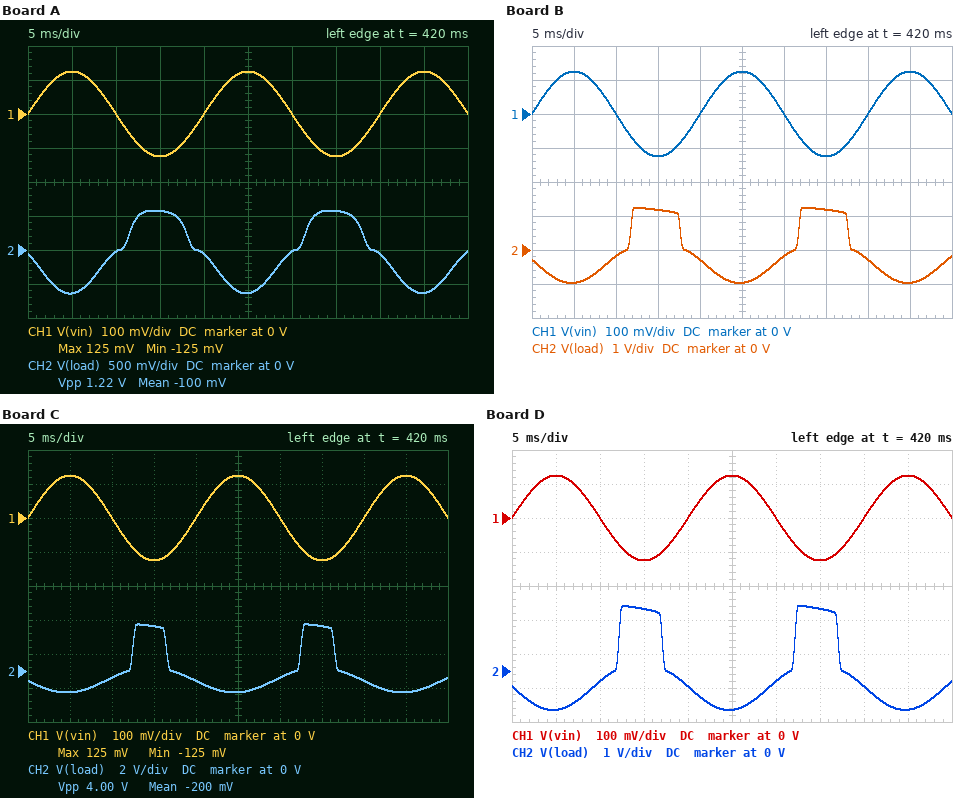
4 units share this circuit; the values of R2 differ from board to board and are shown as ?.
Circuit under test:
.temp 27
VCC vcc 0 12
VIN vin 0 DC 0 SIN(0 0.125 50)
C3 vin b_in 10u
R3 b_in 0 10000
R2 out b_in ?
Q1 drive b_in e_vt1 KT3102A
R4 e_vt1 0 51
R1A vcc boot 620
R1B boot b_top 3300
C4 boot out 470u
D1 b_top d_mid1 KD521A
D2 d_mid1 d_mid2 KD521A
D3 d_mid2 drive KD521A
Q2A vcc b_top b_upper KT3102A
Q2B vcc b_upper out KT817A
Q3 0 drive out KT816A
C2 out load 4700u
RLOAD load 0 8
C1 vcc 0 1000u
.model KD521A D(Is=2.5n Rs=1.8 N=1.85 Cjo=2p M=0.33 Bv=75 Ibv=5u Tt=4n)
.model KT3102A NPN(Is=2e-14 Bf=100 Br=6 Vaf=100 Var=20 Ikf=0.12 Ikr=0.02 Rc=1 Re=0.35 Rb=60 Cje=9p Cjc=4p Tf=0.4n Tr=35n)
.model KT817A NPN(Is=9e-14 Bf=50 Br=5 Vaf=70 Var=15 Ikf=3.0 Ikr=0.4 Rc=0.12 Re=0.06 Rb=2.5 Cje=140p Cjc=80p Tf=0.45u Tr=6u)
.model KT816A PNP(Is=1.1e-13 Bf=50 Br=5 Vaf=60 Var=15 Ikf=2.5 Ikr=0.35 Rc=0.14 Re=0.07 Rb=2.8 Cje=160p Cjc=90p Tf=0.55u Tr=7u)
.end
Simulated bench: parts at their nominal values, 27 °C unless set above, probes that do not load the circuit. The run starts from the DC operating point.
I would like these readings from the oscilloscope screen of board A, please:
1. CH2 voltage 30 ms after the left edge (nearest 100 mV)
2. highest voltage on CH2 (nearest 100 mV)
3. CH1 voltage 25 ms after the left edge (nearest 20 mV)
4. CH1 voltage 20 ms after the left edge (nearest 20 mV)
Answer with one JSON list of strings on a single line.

["0 V", "600 mV", "120 mV", "0 V"]
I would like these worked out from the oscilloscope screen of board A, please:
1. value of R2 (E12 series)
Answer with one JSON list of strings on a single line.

["150 kΩ"]
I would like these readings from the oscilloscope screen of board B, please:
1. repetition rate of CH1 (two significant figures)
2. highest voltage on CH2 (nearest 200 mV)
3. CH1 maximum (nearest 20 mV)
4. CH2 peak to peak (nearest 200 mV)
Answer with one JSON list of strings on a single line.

["50 Hz", "1.2 V", "120 mV", "2.2 V"]
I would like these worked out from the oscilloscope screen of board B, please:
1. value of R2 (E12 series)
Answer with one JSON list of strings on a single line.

["120 kΩ"]
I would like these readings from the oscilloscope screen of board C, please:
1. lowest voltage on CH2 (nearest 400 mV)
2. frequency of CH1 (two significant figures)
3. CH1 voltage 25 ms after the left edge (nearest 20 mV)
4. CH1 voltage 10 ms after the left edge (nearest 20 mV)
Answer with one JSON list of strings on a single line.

["-1.2 V", "50 Hz", "120 mV", "0 V"]
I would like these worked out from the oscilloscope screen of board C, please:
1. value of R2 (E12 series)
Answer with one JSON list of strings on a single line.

["82 kΩ"]
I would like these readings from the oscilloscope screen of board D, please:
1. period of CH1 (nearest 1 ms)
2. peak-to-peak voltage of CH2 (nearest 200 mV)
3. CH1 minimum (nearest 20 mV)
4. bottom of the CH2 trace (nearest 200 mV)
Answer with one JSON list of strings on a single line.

["20 ms", "3.0 V", "-120 mV", "-1.2 V"]
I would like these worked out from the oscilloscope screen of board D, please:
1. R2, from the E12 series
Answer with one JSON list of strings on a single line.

["100 kΩ"]
